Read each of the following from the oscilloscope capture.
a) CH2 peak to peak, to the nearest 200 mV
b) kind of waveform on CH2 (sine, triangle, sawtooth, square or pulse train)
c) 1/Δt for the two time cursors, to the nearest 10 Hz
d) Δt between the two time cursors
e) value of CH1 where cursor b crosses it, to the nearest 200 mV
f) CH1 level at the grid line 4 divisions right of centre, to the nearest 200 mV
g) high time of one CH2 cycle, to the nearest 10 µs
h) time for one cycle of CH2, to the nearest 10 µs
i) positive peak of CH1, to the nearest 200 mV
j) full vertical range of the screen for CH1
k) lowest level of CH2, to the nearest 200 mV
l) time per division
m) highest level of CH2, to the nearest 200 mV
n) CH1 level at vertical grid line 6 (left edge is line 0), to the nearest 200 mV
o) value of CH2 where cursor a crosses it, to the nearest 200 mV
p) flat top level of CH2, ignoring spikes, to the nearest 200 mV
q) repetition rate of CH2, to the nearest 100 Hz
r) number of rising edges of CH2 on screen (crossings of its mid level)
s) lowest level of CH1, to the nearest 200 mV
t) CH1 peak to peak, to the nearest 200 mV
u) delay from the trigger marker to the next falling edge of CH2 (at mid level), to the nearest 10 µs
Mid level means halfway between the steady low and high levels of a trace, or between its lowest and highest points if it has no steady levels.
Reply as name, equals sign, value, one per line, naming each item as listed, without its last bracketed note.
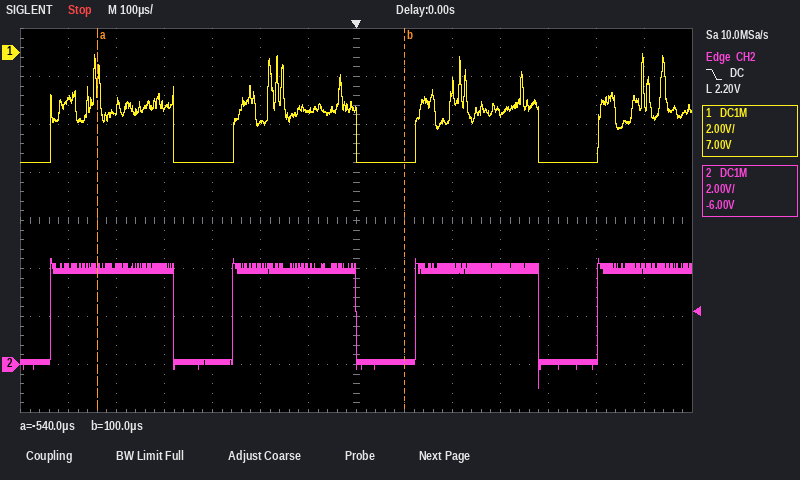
CH2 peak to peak, to the nearest 200 mV = 5.4 V
kind of waveform on CH2 = pulse train
1/Δt for the two time cursors, to the nearest 10 Hz = 1.56 kHz
Δt between the two time cursors = 640 µs
value of CH1 where cursor b crosses it, to the nearest 200 mV = -4.6 V
CH1 level at the grid line 4 divisions right of centre, to the nearest 200 mV = -4.6 V
high time of one CH2 cycle, to the nearest 10 µs = 260 µs
time for one cycle of CH2, to the nearest 10 µs = 380 µs
positive peak of CH1, to the nearest 200 mV = 0.0 V
full vertical range of the screen for CH1 = 16 V
lowest level of CH2, to the nearest 200 mV = -1.0 V
time per division = 100 µs
highest level of CH2, to the nearest 200 mV = 4.4 V
CH1 level at vertical grid line 6 (left edge is line 0), to the nearest 200 mV = -2.4 V
value of CH2 where cursor a crosses it, to the nearest 200 mV = 4.0 V
flat top level of CH2, ignoring spikes, to the nearest 200 mV = 4.0 V
repetition rate of CH2, to the nearest 100 Hz = 2.6 kHz
number of rising edges of CH2 on screen = 4
lowest level of CH1, to the nearest 200 mV = -4.6 V
CH1 peak to peak, to the nearest 200 mV = 4.6 V
delay from the trigger marker to the next falling edge of CH2 (at mid level), to the nearest 10 µs = 380 µs
